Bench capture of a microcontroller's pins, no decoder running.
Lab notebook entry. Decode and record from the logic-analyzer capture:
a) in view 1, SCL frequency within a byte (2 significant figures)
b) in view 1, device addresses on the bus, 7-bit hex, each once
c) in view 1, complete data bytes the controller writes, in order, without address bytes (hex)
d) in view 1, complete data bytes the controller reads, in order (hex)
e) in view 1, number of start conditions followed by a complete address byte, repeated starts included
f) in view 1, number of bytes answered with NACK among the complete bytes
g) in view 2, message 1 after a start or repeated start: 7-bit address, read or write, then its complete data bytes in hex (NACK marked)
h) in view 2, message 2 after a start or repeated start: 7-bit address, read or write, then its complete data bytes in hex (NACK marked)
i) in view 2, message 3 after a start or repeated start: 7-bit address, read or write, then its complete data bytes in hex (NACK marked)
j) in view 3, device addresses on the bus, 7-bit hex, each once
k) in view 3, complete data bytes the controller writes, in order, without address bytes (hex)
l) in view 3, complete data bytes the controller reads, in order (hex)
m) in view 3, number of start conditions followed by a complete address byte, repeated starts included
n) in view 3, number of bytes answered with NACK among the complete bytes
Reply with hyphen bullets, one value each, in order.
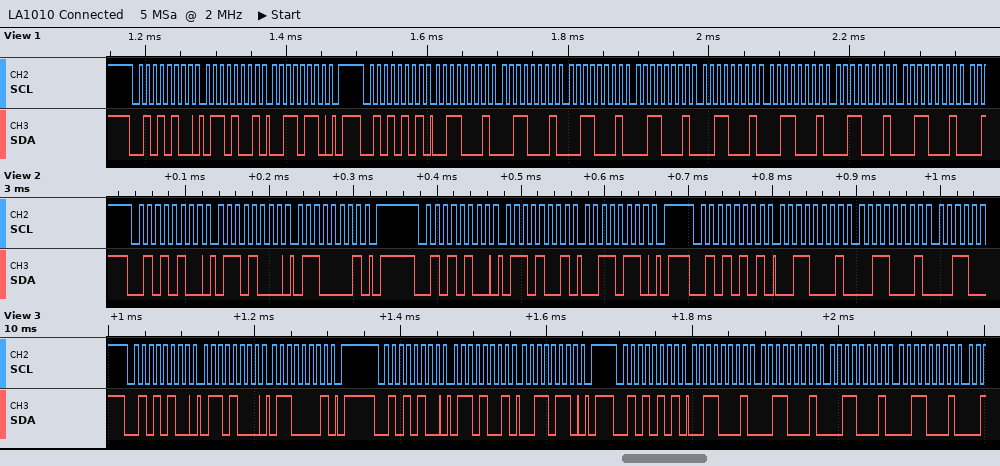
- 100 kHz
- 0x2A
- 69 36
- 31 31 31 31 31 31 31 31
- 2
- 0
- 0x2A write: 68 61
- 0x2A write: 69 36
- 0x2A read: 31 31
- 0x2A
- 68 61 69 36
- 31 31 31 31
- 3
- 0
